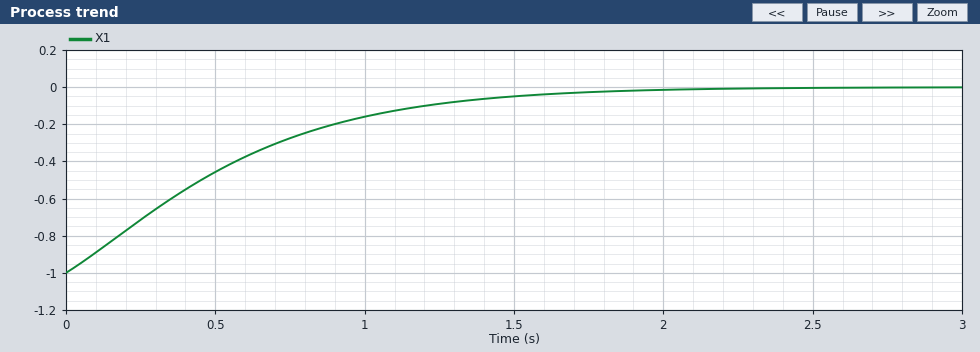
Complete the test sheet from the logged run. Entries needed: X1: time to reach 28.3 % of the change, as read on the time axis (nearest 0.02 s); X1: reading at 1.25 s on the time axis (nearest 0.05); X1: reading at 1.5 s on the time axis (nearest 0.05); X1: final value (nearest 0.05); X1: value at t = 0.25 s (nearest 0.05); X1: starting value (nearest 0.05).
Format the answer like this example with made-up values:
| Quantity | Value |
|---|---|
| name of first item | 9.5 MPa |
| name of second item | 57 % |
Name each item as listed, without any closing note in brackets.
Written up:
| Quantity | Value |
|---|---|
| X1: time to reach 28.3 % of the change, as read on the time axis | 0.24 s |
| X1: reading at 1.25 s on the time axis | -0.10 |
| X1: reading at 1.5 s on the time axis | -0.05 |
| X1: final value | 0.00 |
| X1: value at t = 0.25 s | -0.70 |
| X1: starting value | -1.00 |
